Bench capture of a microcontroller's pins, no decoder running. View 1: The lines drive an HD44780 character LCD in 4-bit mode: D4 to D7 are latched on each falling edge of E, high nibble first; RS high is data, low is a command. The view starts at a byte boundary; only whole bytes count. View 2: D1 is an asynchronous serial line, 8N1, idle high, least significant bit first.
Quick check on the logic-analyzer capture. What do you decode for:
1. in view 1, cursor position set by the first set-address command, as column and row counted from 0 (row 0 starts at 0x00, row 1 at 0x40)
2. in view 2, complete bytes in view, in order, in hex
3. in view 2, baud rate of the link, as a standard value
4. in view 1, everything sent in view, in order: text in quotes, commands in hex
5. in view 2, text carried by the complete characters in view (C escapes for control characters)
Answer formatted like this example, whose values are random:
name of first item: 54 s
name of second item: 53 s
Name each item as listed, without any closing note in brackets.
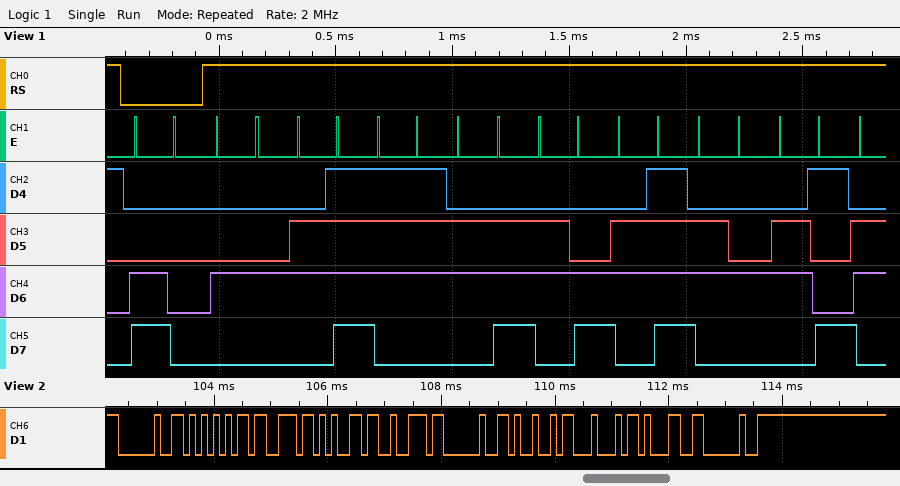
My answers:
in view 1, cursor position set by the first set-address command, as column and row counted from 0: column 0, row 1
in view 2, complete bytes in view, in order, in hex: 0x20 0x55 0x73 0x65 0x72 0x20 0x49 0x44 0x31 0x20
in view 2, baud rate of the link, as a standard value: 9600 baud
in view 1, everything sent in view, in order: text in quotes, commands in hex: 0xC0 "Downlodi"
in view 2, text carried by the complete characters in view: " User ID1 "
